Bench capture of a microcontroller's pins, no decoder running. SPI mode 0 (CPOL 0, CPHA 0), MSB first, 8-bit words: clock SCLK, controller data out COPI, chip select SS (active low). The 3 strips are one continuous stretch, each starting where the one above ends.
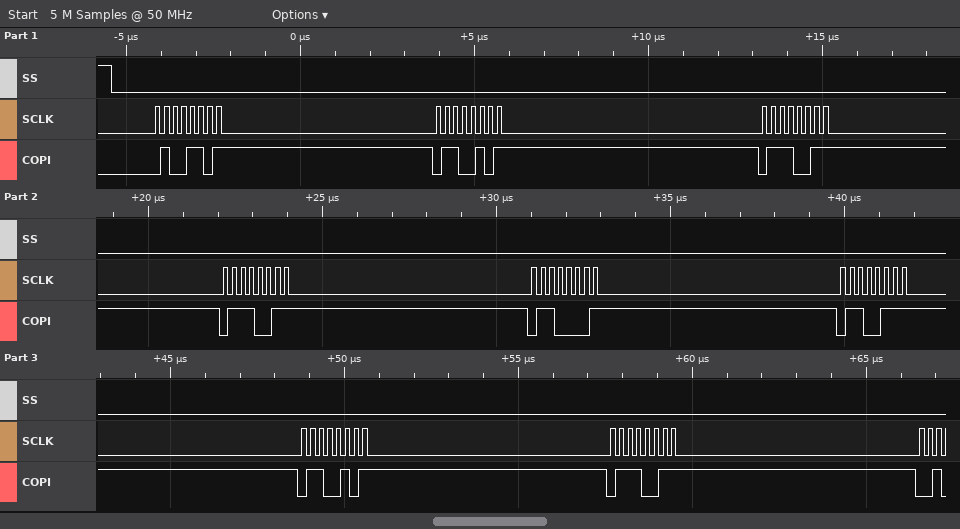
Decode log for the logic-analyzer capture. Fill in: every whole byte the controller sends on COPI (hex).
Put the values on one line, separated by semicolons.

4D 65 73 73 61 67 65 73
